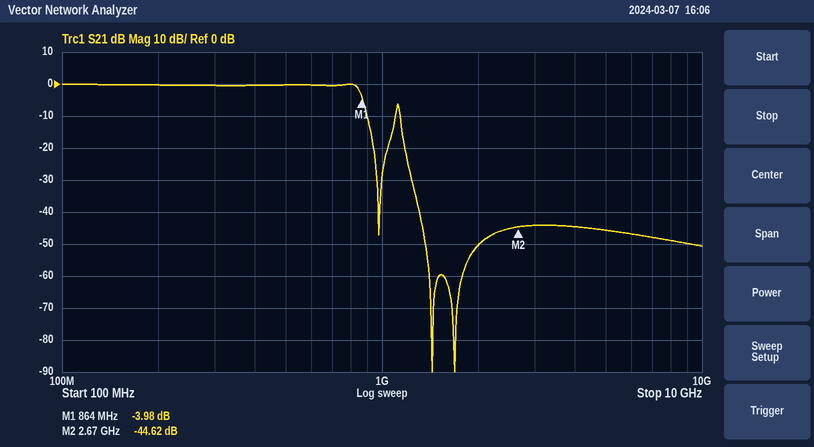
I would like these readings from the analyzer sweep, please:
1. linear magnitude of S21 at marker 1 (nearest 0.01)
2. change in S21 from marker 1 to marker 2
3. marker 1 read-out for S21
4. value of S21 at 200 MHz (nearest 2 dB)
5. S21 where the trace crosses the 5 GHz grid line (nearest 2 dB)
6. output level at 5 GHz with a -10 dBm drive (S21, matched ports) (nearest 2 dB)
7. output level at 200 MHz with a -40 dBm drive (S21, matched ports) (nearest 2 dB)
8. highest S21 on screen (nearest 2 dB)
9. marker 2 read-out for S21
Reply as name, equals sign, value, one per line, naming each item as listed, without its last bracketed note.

linear magnitude of S21 at marker 1 = 0.63
change in S21 from marker 1 to marker 2 = -40.64 dB
marker 1 read-out for S21 = -3.98 dB
value of S21 at 200 MHz = 0 dB
S21 where the trace crosses the 5 GHz grid line = -46 dB
output level at 5 GHz with a -10 dBm drive (S21, matched ports) = -56 dBm
output level at 200 MHz with a -40 dBm drive (S21, matched ports) = -40 dBm
highest S21 on screen = 0 dB
marker 2 read-out for S21 = -44.62 dB
